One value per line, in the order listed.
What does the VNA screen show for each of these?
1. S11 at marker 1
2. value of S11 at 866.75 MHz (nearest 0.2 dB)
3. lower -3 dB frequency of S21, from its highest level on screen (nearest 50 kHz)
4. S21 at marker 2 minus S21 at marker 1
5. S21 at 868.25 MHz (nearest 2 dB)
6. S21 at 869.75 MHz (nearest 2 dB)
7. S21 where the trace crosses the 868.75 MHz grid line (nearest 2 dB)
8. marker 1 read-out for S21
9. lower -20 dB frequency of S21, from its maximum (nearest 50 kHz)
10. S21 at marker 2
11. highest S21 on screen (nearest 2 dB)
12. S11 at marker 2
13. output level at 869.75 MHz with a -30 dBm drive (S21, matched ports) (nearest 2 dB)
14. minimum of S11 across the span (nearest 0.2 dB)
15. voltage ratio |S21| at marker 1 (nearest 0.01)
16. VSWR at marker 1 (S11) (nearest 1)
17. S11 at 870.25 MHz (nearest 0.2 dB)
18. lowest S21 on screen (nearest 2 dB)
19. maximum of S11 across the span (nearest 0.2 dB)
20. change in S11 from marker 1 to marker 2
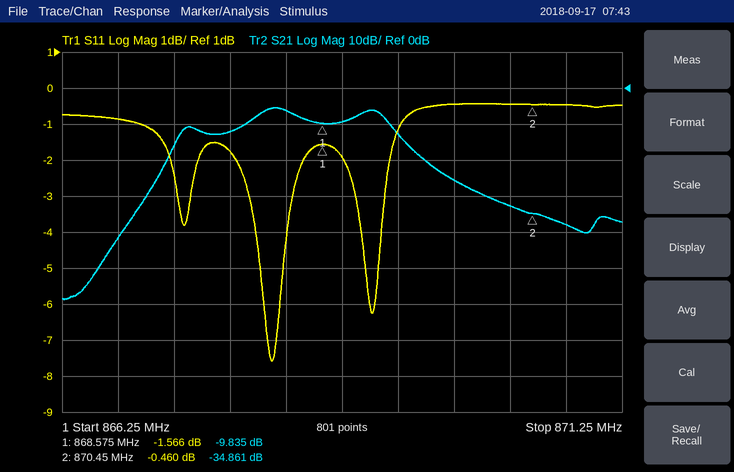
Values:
-1.566 dB
-0.8 dB
867.95 MHz
-25.026 dB
-6 dB
-26 dB
-10 dB
-9.835 dB
867.10 MHz
-34.861 dB
-6 dB
-0.460 dB
-56 dBm
-7.6 dB
0.32
11
-0.4 dB
-58 dB
-0.4 dB
1.106 dB
